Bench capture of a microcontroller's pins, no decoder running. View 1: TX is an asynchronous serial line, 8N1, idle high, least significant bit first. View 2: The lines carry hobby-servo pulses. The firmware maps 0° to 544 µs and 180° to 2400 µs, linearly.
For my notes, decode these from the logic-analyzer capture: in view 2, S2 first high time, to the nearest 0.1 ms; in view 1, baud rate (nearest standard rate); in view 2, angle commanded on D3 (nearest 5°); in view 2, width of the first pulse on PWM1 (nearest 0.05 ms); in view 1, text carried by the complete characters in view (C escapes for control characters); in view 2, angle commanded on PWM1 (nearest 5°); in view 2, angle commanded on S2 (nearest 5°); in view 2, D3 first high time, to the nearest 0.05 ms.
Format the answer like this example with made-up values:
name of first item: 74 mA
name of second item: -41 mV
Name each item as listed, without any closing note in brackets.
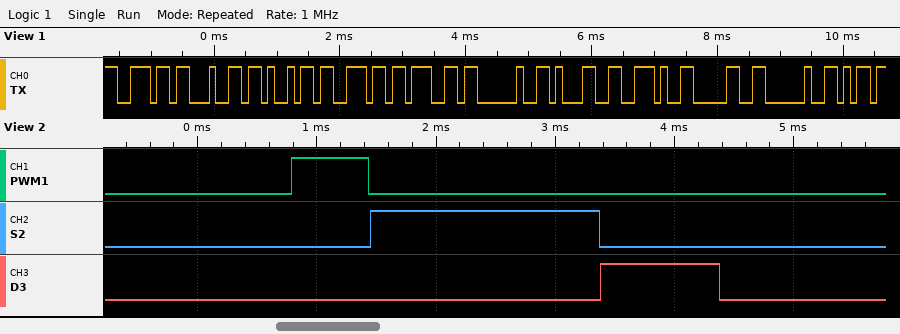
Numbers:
in view 2, S2 first high time, to the nearest 0.1 ms: 1.9 ms
in view 1, baud rate: 9600 baud
in view 2, angle commanded on D3: 45°
in view 2, width of the first pulse on PWM1: 0.65 ms
in view 1, text carried by the complete characters in view: "nding 1.0 "
in view 2, angle commanded on PWM1: 10°
in view 2, angle commanded on S2: 135°
in view 2, D3 first high time, to the nearest 0.05 ms: 1.00 ms
